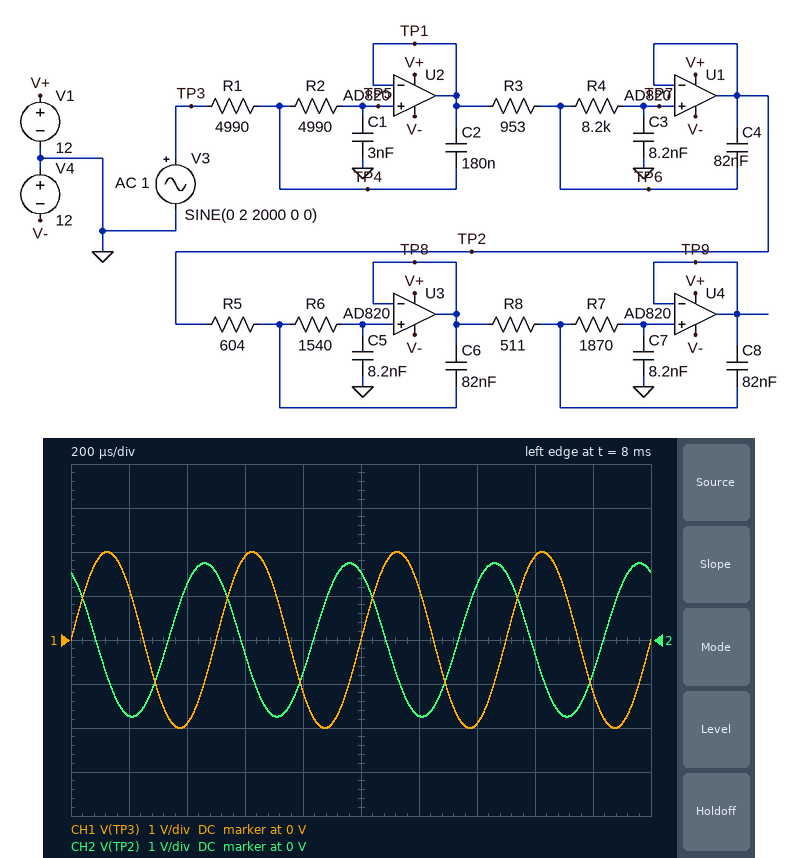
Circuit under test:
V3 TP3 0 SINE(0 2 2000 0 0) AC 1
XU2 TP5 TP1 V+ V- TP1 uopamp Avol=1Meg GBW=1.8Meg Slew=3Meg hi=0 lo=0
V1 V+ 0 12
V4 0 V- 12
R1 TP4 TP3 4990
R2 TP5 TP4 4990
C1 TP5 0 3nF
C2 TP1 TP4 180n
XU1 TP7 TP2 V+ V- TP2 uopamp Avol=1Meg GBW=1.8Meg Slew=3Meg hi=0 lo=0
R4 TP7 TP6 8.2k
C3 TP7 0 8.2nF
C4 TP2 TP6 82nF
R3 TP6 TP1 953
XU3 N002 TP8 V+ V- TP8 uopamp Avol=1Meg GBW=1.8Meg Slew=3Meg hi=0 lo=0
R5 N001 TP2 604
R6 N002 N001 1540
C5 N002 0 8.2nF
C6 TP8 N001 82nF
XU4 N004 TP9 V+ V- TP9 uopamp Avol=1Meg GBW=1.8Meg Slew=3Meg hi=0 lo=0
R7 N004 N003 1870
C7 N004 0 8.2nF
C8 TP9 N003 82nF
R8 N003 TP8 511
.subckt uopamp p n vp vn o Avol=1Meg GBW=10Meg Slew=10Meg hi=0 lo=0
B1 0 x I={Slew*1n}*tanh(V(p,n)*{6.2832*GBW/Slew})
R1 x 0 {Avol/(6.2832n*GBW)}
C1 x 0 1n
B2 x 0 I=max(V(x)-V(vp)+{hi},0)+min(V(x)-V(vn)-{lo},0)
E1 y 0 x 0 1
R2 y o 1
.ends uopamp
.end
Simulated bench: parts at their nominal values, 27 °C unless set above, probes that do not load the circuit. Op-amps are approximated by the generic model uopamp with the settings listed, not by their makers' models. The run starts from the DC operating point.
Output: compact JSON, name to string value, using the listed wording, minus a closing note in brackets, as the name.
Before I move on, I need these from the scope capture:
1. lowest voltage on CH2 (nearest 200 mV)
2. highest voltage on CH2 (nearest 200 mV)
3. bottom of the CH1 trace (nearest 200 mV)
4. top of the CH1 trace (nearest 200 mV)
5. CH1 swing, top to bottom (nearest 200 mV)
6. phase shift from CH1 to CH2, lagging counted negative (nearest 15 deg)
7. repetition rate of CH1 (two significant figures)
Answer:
{"lowest voltage on CH2": "-1.8 V", "highest voltage on CH2": "1.8 V", "bottom of the CH1 trace": "-2.0 V", "top of the CH1 trace": "2.0 V", "CH1 swing, top to bottom": "4.0 V", "phase shift from CH1 to CH2, lagging counted negative": "120 deg", "repetition rate of CH1": "2.0 kHz"}
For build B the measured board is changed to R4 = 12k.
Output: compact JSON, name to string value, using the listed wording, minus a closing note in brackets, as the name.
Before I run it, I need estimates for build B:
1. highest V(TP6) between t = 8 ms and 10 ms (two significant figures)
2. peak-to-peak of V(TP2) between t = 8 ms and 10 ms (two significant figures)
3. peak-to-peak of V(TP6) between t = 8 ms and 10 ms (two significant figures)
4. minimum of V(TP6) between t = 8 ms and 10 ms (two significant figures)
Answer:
{"highest V(TP6) between t = 8 ms and 10 ms": "2.0 V", "peak-to-peak of V(TP2) between t = 8 ms and 10 ms": "2.5 V", "peak-to-peak of V(TP6) between t = 8 ms and 10 ms": "3.9 V", "minimum of V(TP6) between t = 8 ms and 10 ms": "-2.0 V"}
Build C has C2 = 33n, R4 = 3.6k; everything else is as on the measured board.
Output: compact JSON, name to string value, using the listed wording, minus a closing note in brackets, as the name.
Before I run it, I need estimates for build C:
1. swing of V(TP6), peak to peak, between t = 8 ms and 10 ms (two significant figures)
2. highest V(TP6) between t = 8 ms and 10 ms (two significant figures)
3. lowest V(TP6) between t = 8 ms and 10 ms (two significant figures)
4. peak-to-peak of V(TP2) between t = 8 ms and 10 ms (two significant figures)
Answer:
{"swing of V(TP6), peak to peak, between t = 8 ms and 10 ms": "7.6 V", "highest V(TP6) between t = 8 ms and 10 ms": "3.8 V", "lowest V(TP6) between t = 8 ms and 10 ms": "-3.8 V", "peak-to-peak of V(TP2) between t = 8 ms and 10 ms": "7.1 V"}
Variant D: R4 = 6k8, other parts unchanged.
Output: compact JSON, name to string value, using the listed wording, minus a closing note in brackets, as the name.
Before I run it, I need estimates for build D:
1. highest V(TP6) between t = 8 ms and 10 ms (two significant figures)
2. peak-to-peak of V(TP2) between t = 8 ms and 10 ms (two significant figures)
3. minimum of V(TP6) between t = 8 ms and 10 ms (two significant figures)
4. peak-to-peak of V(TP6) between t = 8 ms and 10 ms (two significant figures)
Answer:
{"highest V(TP6) between t = 8 ms and 10 ms": "2.4 V", "peak-to-peak of V(TP2) between t = 8 ms and 10 ms": "3.9 V", "minimum of V(TP6) between t = 8 ms and 10 ms": "-2.4 V", "peak-to-peak of V(TP6) between t = 8 ms and 10 ms": "4.8 V"}
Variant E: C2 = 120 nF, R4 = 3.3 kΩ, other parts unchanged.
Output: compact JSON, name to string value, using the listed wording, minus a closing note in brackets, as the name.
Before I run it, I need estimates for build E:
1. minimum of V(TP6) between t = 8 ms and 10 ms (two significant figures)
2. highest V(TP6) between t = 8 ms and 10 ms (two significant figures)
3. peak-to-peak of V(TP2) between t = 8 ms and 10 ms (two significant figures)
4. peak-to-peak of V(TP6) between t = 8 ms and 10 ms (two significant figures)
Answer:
{"minimum of V(TP6) between t = 8 ms and 10 ms": "-4.7 V", "highest V(TP6) between t = 8 ms and 10 ms": "4.7 V", "peak-to-peak of V(TP2) between t = 8 ms and 10 ms": "8.9 V", "peak-to-peak of V(TP6) between t = 8 ms and 10 ms": "9.4 V"}
